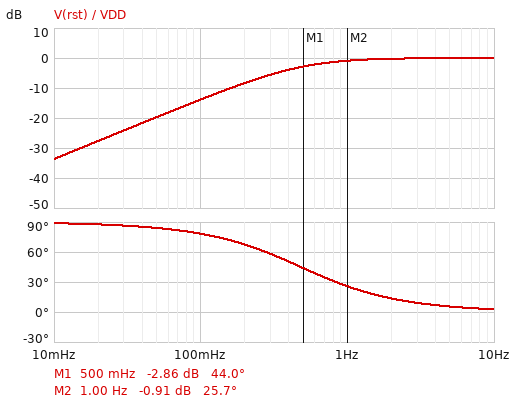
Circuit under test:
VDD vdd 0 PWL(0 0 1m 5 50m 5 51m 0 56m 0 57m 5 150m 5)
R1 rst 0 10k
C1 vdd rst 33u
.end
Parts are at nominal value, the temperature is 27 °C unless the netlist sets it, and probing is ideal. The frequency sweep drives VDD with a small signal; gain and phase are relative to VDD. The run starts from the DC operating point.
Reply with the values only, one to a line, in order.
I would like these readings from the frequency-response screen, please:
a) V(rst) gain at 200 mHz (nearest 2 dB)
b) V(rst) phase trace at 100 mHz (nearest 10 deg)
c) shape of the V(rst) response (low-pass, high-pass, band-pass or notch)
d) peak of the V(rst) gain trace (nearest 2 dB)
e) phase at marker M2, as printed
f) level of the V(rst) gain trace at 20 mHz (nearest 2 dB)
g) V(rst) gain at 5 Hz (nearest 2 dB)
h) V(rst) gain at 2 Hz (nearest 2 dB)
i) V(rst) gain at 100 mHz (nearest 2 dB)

-8 dB
80 deg
high-pass
0 dB
25.7 deg
-28 dB
0 dB
0 dB
-14 dB
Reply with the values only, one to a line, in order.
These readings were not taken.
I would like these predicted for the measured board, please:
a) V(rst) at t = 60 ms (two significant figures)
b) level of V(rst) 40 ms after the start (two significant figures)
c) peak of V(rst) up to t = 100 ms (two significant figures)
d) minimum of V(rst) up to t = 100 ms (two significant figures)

4.3 V
4.4 V
5.0 V
-700 mV
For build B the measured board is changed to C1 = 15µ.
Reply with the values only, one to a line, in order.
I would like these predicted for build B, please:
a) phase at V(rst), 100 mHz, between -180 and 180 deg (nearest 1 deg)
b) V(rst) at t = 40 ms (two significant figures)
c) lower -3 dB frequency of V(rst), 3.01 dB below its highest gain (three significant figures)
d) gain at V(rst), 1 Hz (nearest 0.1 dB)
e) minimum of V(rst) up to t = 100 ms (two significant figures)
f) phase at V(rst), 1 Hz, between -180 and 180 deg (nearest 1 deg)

85 deg
3.8 V
1.06 Hz
-3.3 dB
-1.4 V
47 deg
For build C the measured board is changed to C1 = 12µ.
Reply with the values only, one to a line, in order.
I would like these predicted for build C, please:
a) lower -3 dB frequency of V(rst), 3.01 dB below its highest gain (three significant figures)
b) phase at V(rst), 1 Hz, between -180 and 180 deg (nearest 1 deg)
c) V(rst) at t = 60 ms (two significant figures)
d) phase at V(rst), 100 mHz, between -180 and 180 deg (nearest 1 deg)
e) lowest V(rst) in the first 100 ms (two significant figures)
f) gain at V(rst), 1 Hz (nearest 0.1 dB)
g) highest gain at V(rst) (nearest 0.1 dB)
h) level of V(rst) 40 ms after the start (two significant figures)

1.33 Hz
53 deg
3.3 V
86 deg
-1.7 V
-4.4 dB
0 dB
3.6 V
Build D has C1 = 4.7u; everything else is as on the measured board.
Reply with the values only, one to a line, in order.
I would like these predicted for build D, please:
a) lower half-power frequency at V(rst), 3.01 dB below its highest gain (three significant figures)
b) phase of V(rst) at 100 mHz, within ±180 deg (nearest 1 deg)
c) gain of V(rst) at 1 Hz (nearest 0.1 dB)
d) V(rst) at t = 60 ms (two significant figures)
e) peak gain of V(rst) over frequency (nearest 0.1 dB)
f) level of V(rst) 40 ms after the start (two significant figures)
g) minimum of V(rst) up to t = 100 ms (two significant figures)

3.39 Hz
88 deg
-11.0 dB
2.0 V
0 dB
2.2 V
-3.2 V
